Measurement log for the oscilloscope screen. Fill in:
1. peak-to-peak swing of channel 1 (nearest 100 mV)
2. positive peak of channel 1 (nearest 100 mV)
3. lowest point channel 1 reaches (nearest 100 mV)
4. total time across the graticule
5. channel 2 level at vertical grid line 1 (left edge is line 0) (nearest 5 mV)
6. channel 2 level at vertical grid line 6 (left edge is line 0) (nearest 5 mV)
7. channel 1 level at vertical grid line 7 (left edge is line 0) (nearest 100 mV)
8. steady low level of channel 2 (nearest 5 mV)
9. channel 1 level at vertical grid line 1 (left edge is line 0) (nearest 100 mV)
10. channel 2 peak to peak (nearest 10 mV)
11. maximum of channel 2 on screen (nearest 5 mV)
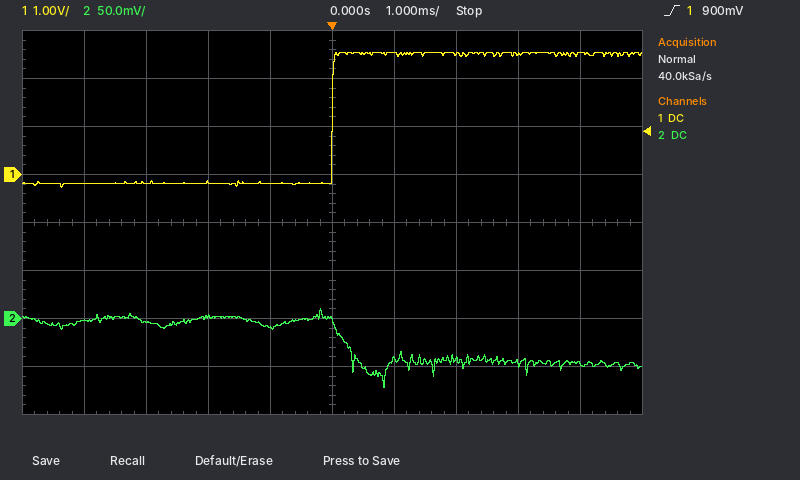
2.8 V
2.5 V
-300 mV
10 ms
0 mV
-45 mV
2.5 V
-45 mV
-200 mV
80 mV
10 mV
